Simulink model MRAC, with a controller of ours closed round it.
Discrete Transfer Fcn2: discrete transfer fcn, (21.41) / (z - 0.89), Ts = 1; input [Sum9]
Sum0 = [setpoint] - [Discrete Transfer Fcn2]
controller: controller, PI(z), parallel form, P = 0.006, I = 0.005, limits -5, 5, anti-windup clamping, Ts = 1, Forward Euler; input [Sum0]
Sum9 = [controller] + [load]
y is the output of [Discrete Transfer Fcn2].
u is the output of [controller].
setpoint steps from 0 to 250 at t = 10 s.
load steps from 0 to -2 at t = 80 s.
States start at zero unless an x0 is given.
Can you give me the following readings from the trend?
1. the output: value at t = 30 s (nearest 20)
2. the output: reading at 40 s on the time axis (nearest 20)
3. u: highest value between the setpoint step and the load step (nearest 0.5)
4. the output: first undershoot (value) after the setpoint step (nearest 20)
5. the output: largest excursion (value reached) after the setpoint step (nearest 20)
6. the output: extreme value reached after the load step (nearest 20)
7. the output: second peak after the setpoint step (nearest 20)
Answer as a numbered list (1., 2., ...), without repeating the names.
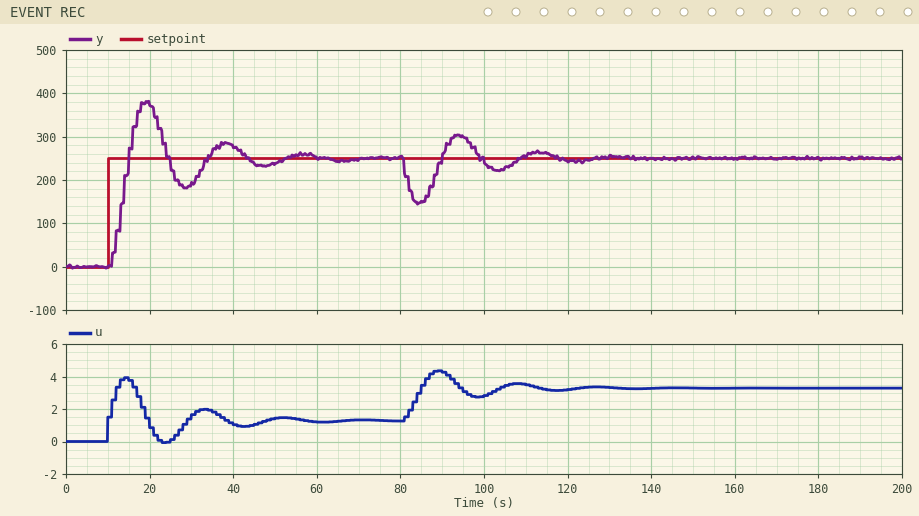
1. 200
2. 280
3. 4.0
4. 180
5. 380
6. 140
7. 280
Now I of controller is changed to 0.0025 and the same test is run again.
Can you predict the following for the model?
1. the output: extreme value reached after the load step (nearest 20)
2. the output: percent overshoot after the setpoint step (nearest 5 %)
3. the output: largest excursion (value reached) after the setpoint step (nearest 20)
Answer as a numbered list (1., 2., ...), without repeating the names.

1. 140
2. 25 %
3. 320
